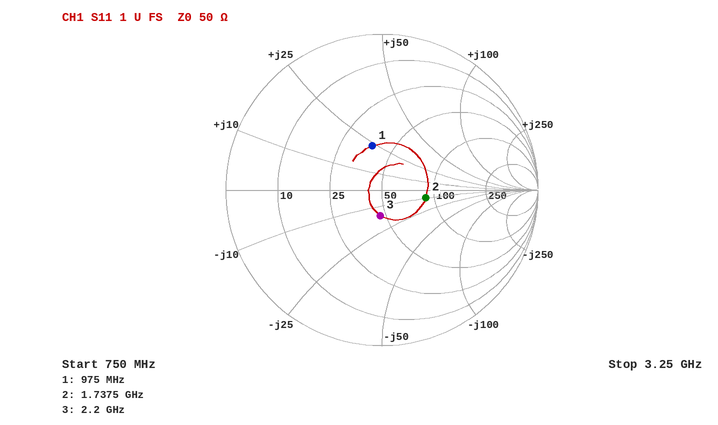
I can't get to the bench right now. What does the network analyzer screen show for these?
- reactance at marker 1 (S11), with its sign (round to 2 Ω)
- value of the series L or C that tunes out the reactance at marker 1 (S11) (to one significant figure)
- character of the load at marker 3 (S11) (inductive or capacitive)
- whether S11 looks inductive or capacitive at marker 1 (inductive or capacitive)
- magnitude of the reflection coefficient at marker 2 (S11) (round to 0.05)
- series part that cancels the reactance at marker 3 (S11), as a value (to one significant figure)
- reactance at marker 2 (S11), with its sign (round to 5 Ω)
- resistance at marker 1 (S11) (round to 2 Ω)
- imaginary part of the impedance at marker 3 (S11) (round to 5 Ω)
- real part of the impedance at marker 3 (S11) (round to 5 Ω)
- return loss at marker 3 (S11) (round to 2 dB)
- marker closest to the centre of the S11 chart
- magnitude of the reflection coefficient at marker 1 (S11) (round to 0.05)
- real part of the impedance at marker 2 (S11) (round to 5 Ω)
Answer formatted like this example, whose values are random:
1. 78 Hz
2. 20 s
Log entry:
1. +24 Ω
2. 7 pF
3. capacitive
4. inductive
5. 0.30
6. 1 nH
7. -10 Ω
8. 38 Ω
9. -15 Ω
10. 45 Ω
11. 16 dB
12. marker 3
13. 0.30
14. 90 Ω
